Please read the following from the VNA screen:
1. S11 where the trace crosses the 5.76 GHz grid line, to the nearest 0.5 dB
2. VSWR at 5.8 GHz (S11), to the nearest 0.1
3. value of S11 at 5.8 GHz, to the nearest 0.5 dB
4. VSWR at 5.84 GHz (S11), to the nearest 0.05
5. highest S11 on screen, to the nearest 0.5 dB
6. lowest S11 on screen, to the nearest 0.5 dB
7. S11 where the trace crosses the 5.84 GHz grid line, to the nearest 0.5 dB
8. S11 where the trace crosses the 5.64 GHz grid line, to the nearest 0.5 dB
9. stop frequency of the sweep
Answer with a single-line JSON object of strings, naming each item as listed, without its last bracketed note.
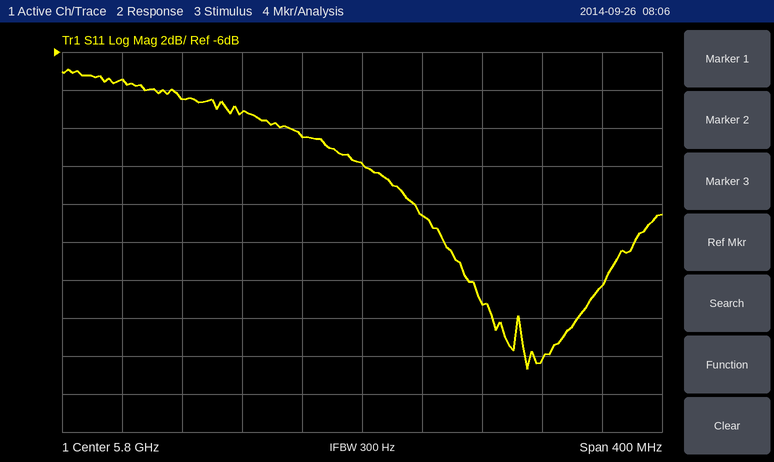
{"S11 where the trace crosses the 5.76 GHz grid line, to the nearest 0.5 dB": "-10.5 dB", "VSWR at 5.8 GHz (S11), to the nearest 0.1": "1.7", "value of S11 at 5.8 GHz, to the nearest 0.5 dB": "-12.0 dB", "VSWR at 5.84 GHz (S11), to the nearest 0.05": "1.45", "highest S11 on screen, to the nearest 0.5 dB": "-7.0 dB", "lowest S11 on screen, to the nearest 0.5 dB": "-22.5 dB", "S11 where the trace crosses the 5.84 GHz grid line, to the nearest 0.5 dB": "-14.5 dB", "S11 where the trace crosses the 5.64 GHz grid line, to the nearest 0.5 dB": "-7.5 dB", "stop frequency of the sweep": "6 GHz"}
